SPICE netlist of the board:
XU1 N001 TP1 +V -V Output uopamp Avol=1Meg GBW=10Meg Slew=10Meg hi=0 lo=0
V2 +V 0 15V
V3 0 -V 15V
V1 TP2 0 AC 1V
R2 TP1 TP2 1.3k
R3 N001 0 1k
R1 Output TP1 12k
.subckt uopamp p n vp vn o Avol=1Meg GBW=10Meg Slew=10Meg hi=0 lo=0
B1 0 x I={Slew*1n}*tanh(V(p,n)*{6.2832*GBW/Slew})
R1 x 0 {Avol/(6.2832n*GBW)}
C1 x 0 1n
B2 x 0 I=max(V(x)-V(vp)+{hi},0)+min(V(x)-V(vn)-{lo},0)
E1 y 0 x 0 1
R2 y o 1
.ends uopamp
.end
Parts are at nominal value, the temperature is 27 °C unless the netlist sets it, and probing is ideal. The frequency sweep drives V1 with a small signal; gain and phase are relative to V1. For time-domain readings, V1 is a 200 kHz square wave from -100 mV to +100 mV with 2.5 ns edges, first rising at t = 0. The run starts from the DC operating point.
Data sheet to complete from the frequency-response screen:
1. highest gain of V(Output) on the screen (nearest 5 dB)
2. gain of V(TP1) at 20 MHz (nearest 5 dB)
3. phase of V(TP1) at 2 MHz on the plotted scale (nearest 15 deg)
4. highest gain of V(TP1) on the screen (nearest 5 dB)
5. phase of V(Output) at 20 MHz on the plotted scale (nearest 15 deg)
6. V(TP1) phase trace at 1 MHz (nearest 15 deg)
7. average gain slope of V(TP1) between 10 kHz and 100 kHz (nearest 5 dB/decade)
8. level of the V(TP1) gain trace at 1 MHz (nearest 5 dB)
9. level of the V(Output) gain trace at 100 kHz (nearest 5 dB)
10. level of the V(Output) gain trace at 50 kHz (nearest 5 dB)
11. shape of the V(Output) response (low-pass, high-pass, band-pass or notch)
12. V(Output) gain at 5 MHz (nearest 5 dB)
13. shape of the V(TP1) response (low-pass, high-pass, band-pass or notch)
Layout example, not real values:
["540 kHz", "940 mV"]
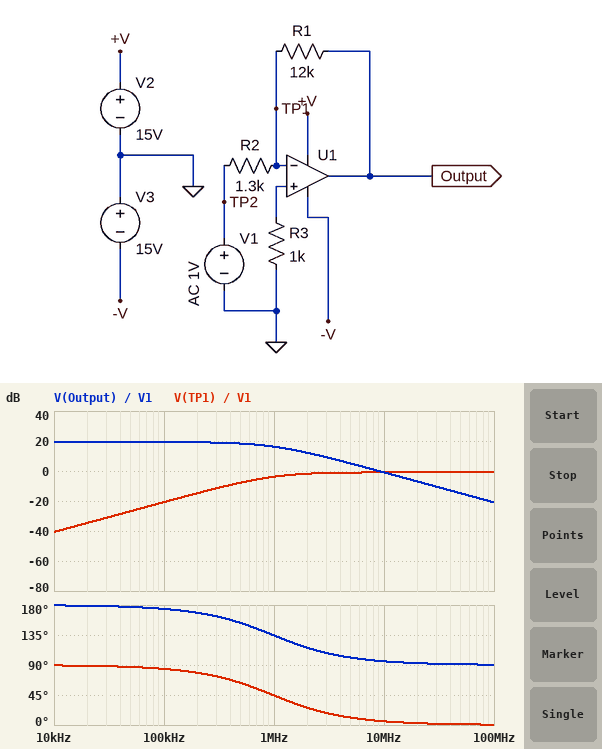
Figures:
["20 dB", "0 dB", "30 deg", "0 dB", "90 deg", "45 deg", "20 dB/decade", "-5 dB", "20 dB", "20 dB", "low-pass", "5 dB", "high-pass"]
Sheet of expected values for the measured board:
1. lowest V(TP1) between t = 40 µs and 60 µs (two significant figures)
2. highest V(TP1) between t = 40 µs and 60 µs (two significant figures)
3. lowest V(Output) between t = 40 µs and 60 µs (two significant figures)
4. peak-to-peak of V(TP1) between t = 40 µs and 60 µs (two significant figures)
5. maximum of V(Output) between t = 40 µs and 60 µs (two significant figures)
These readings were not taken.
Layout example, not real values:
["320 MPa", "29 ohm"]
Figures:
["-180 mV", "180 mV", "-920 mV", "360 mV", "920 mV"]
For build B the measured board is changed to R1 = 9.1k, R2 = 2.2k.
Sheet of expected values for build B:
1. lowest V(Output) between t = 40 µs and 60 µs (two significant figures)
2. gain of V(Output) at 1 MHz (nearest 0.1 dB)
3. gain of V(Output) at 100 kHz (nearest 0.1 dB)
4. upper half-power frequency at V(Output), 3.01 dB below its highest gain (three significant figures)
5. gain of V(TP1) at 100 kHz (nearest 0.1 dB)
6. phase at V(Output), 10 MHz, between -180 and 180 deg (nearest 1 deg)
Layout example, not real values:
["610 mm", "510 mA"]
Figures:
["-410 mV", "11.3 dB", "12.3 dB", "1.95 MHz", "-27.7 dB", "101 deg"]
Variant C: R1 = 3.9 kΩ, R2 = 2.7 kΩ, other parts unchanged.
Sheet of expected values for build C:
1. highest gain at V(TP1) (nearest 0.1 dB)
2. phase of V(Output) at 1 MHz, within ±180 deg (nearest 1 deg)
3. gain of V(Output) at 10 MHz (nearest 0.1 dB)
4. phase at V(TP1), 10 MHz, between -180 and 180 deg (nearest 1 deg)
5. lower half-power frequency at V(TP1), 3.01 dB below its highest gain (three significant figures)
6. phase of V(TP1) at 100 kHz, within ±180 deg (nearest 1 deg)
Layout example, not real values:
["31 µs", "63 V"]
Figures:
["-4.6 dB", "166 deg", "-5.2 dB", "22 deg", "4.09 MHz", "89 deg"]
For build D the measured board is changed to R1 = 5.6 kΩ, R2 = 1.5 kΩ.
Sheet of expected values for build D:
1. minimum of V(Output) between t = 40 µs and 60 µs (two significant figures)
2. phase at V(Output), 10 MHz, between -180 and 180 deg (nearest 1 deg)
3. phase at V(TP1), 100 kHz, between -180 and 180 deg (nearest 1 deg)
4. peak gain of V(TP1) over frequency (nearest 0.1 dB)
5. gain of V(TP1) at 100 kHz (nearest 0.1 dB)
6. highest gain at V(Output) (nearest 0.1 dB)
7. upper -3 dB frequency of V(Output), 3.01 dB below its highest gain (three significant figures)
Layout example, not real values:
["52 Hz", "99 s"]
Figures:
["-370 mV", "102 deg", "87 deg", "-2.1 dB", "-28.6 dB", "11.4 dB", "2.11 MHz"]
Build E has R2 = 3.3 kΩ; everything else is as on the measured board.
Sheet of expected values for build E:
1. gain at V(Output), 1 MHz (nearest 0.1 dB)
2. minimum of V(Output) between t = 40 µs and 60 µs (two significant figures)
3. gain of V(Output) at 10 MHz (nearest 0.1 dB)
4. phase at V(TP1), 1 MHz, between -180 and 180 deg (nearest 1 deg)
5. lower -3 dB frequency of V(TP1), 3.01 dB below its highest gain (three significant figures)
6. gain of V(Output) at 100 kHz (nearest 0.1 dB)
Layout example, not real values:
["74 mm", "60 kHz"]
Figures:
["10.4 dB", "-360 mV", "-2.3 dB", "65 deg", "2.16 MHz", "11.2 dB"]
